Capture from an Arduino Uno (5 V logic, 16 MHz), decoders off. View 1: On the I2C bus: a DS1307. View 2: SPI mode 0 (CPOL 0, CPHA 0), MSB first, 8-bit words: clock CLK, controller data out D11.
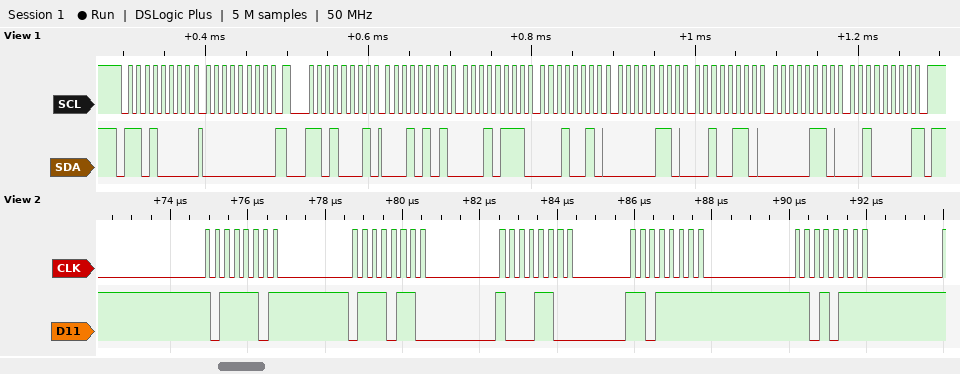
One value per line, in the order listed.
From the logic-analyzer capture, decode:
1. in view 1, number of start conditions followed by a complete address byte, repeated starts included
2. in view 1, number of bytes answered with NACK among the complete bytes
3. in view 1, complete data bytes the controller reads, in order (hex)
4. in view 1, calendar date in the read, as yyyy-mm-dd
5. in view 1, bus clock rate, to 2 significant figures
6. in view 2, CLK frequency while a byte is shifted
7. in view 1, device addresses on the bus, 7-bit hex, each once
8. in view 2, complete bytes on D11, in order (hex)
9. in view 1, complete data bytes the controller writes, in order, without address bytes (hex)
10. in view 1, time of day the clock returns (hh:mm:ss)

2
1
15 17 12 06 26 06 20
2020-06-26
100 kHz
4 MHz
0x68
BD 76 8C DF D7
00
12:17:15
